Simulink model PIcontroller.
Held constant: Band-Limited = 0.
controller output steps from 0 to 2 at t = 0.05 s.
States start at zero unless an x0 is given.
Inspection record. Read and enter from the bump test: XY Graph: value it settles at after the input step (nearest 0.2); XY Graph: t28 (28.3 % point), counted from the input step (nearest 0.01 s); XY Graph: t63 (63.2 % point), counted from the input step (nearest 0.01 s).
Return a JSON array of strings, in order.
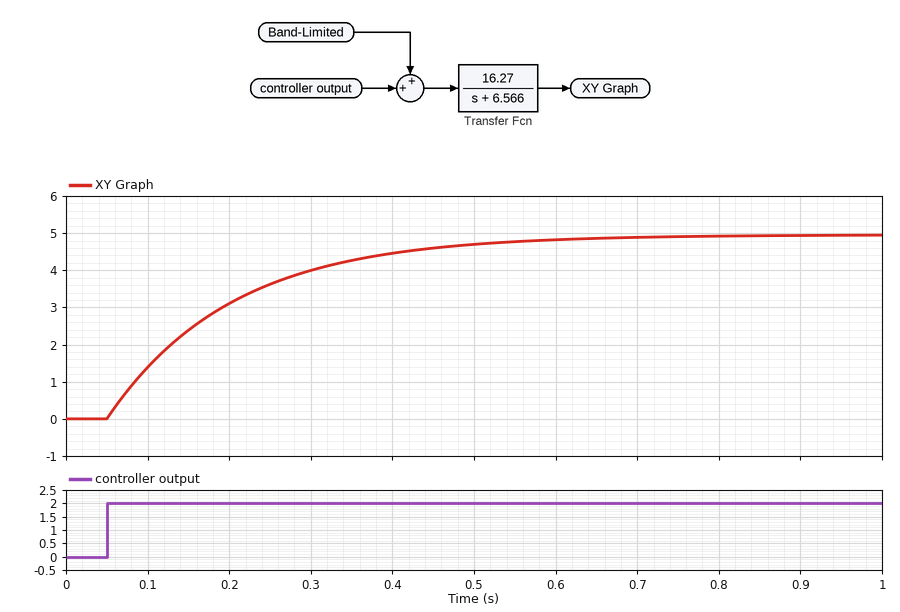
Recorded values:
["5.0", "0.05 s", "0.15 s"]
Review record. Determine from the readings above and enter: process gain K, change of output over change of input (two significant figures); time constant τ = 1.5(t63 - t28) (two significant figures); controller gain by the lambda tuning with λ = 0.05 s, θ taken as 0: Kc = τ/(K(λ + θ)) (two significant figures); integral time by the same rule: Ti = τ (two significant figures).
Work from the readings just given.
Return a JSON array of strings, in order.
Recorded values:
["2.5", "0.15 s", "1.2", "0.15 s"]
